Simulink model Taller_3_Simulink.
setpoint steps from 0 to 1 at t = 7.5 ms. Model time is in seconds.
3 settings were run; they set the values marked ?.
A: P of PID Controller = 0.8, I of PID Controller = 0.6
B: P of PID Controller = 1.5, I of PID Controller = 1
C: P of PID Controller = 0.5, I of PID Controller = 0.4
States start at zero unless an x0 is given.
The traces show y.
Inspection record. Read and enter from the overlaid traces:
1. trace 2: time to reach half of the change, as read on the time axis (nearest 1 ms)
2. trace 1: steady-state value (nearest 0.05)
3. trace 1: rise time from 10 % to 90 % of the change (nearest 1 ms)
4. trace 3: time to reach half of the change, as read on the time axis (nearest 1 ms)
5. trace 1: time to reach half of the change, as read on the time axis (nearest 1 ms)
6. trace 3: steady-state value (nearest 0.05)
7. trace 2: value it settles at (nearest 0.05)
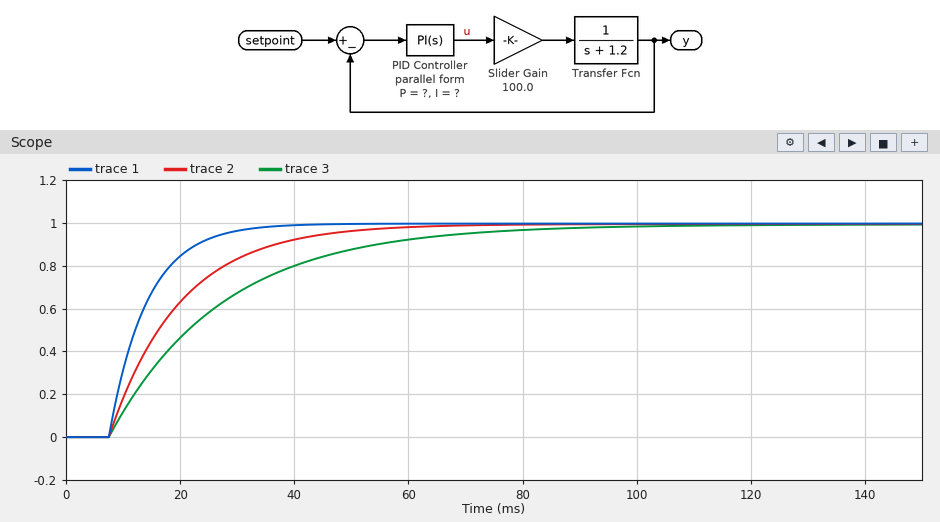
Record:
16 ms
1.00
15 ms
21 ms
12 ms
1.00
1.00
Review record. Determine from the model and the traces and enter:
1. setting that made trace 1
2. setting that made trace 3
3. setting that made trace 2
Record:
B
C
A
